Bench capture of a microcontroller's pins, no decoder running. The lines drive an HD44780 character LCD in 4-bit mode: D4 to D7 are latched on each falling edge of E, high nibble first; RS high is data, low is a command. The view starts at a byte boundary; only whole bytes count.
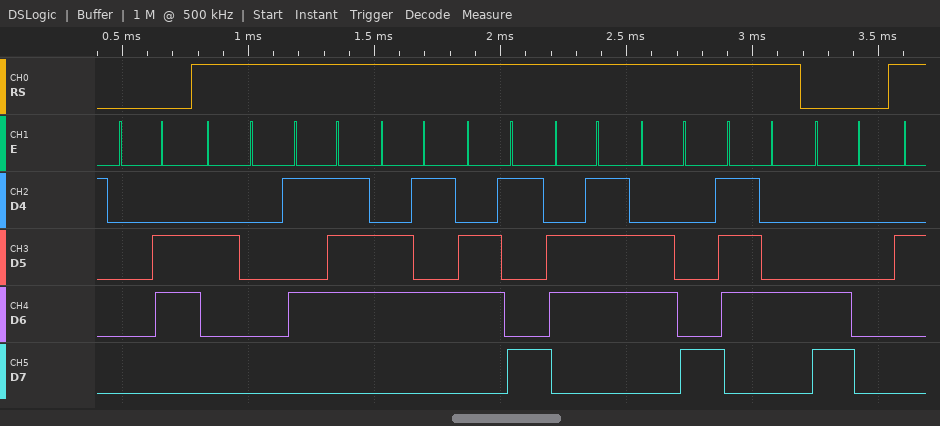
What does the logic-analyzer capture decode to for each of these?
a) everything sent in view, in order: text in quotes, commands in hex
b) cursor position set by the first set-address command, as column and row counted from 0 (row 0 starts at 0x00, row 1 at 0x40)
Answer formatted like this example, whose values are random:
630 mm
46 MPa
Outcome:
0x06 " Weight" 0xC0
column 0, row 1
